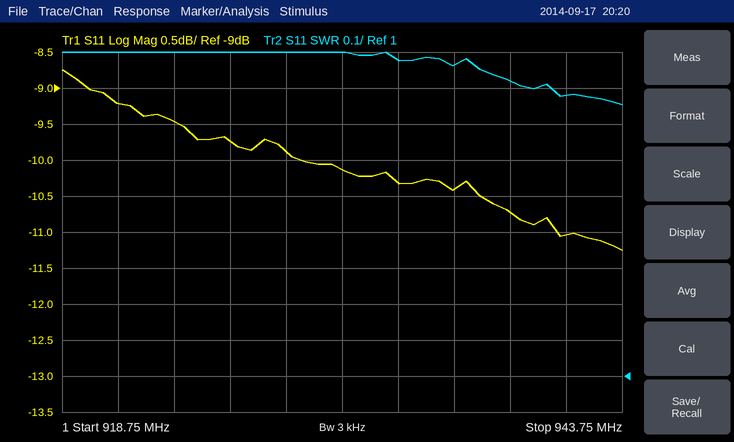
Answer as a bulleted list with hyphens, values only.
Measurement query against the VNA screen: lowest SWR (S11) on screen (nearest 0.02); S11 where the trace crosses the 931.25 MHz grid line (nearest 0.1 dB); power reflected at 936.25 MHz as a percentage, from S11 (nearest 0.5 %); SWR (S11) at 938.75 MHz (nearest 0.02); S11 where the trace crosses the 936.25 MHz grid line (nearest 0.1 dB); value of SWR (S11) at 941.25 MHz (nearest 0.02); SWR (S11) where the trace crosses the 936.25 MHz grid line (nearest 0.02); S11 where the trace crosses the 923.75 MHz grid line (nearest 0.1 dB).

- 1.76
- -10.1 dB
- 9.0 %
- 1.82
- -10.4 dB
- 1.78
- 1.86
- -9.5 dB
